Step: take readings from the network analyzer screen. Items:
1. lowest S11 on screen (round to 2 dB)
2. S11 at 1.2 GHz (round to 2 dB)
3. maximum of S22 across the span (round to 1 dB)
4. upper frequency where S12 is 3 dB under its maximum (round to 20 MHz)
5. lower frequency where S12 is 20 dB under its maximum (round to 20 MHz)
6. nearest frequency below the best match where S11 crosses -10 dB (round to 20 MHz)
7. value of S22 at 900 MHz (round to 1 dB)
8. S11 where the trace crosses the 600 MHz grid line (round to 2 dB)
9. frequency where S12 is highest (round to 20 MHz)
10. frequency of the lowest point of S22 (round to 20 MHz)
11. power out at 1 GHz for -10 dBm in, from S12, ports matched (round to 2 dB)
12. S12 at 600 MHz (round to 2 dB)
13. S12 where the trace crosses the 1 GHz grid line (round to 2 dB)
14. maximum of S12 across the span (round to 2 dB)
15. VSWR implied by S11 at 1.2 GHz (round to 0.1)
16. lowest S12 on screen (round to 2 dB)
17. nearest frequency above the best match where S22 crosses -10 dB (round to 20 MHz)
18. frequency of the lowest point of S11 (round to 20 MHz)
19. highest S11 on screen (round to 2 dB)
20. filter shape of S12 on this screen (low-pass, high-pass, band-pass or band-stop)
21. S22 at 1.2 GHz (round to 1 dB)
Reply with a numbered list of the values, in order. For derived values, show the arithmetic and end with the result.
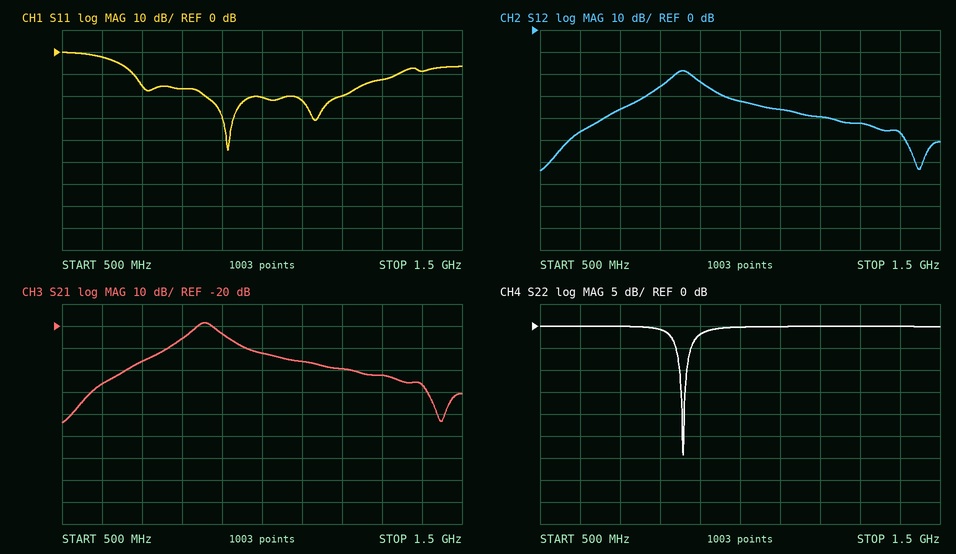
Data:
1. -44 dB
2. -20 dB
3. 0 dB
4. 880 MHz
5. 680 MHz
6. 680 MHz
7. -2 dB
8. -2 dB
9. 860 MHz
10. 860 MHz
11. -10 dBm + (-32 dB) = -42 dBm
12. -46 dB
13. -32 dB
14. -18 dB
15. |Γ| = 10^(-20/20) = 0.1000; VSWR = (1 + 0.1000)/(1 − 0.1000) ≈ 1.2
16. -64 dB
17. 860 MHz
18. 920 MHz
19. 0 dB
20. band-pass
21. 0 dB
